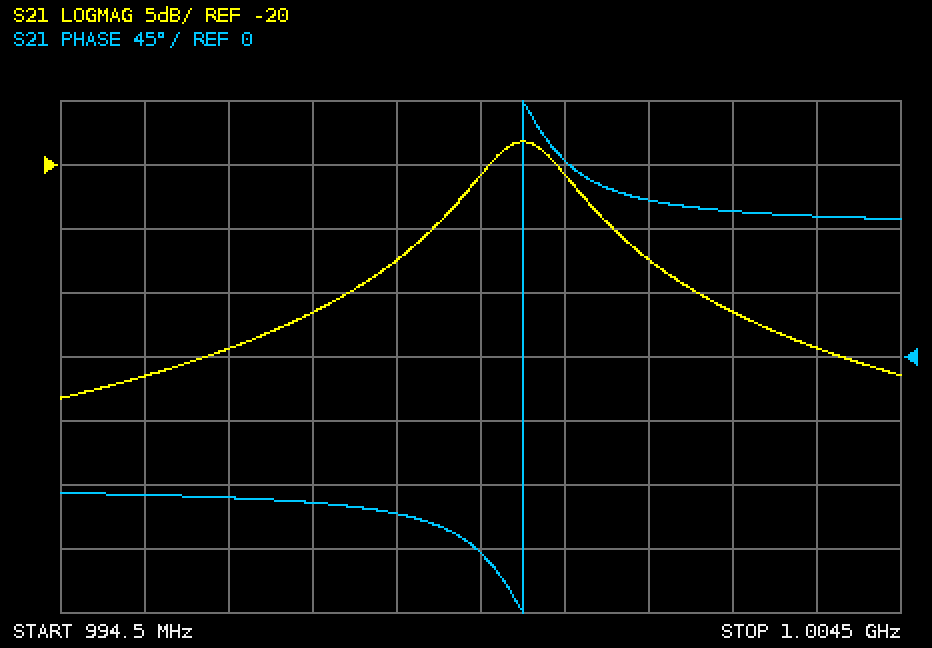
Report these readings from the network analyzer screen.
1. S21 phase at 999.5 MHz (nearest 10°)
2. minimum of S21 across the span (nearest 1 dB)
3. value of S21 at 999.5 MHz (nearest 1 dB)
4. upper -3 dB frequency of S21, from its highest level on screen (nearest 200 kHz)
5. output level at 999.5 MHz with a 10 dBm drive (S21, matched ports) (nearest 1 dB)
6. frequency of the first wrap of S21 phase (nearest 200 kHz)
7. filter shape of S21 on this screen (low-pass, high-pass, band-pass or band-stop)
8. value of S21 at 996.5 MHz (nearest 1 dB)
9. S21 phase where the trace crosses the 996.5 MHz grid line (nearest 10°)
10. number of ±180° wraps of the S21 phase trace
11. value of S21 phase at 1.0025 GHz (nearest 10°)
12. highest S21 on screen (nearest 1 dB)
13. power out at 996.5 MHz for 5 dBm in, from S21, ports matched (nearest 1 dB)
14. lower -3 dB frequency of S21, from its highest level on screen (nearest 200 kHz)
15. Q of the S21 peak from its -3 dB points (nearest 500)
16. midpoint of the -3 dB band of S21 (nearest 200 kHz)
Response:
-140°
-38 dB
-21 dB
1.0006 GHz
-11 dBm
1.0000 GHz
band-pass
-34 dB
-100°
1
100°
-18 dB
-29 dBm
999.4 MHz
1000
1.0000 GHz
